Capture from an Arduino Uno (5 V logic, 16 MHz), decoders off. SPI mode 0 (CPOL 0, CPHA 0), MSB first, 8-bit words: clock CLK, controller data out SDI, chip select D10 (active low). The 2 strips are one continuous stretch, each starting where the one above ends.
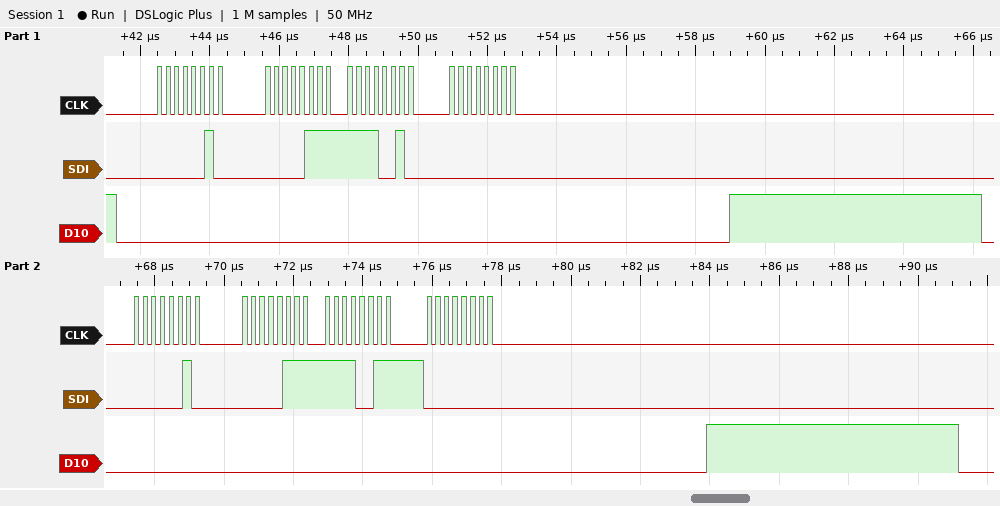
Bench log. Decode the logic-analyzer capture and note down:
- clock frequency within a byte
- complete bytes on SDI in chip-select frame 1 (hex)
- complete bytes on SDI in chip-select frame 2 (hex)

4 MHz
02 07 F2 00
02 07 F3 00
